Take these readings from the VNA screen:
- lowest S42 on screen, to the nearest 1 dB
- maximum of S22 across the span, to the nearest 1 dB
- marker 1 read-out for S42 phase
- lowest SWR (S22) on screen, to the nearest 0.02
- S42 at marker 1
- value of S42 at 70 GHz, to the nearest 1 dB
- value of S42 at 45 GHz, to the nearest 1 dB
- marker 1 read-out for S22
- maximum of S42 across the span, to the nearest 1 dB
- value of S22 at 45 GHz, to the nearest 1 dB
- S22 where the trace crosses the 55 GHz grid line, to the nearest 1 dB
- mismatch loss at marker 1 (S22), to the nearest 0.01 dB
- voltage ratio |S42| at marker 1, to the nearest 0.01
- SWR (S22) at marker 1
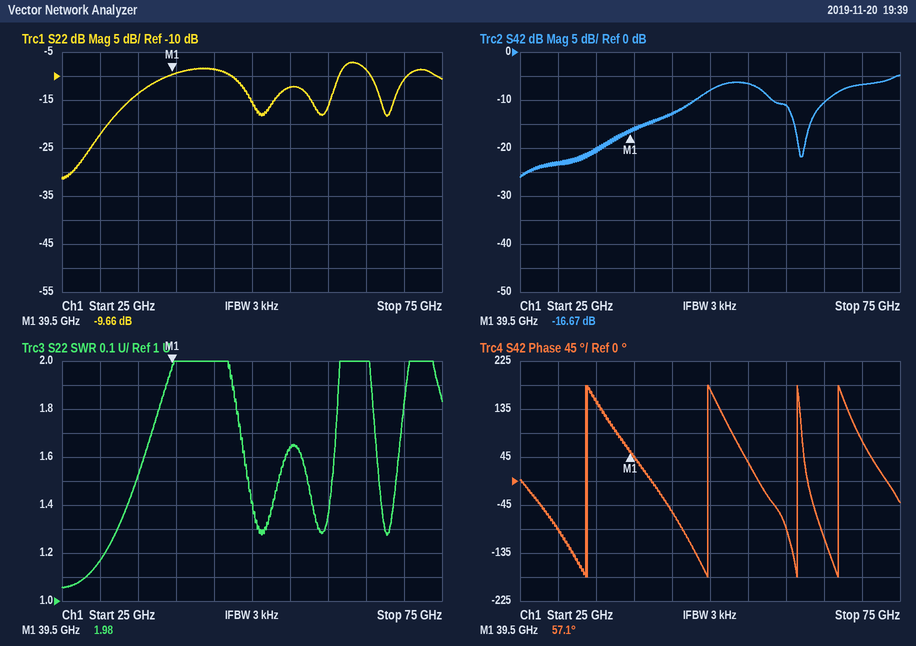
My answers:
-26 dB
-7 dB
57.1°
1.06
-16.67 dB
-7 dB
-13 dB
-9.66 dB
-5 dB
-9 dB
-12 dB
0.50 dB
0.15
1.98
